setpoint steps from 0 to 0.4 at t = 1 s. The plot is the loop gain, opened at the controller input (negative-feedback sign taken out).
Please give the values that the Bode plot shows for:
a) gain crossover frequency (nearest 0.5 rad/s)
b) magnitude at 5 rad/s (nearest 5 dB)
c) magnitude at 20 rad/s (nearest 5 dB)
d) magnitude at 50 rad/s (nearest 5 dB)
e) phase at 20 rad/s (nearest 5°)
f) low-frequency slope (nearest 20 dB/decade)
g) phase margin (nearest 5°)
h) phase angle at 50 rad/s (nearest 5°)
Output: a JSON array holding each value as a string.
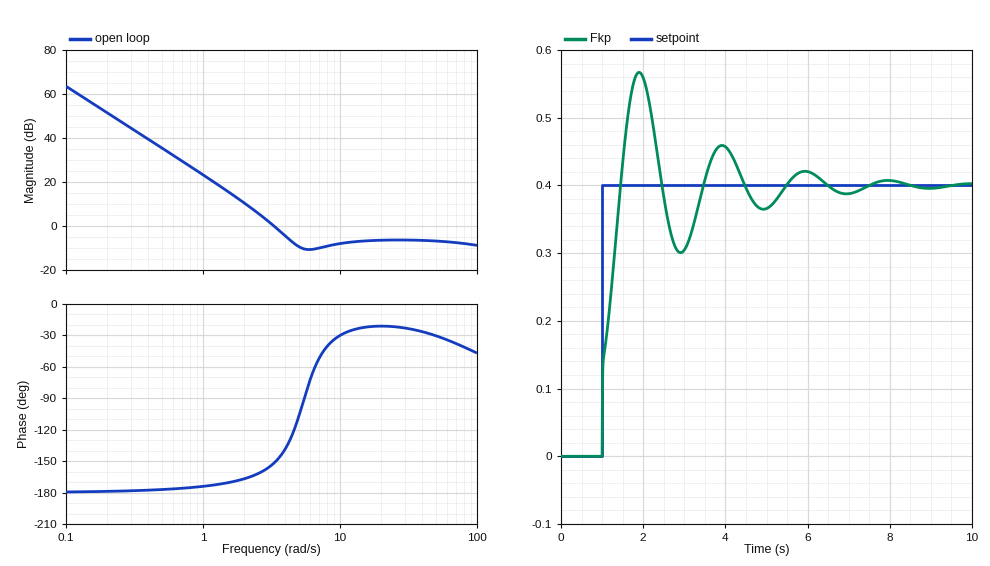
["3.5 rad/s", "-10 dB", "-5 dB", "-5 dB", "-20°", "-40 dB/decade", "30°", "-30°"]
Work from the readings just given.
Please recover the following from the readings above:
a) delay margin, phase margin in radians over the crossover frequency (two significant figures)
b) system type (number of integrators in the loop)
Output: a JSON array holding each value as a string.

["0.15 s", "2"]
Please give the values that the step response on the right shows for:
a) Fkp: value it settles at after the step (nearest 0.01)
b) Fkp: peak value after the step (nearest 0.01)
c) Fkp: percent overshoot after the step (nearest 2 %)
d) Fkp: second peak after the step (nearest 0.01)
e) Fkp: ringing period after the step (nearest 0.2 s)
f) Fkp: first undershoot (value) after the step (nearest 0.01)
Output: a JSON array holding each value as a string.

["0.40", "0.57", "42 %", "0.46", "2.0 s", "0.30"]
